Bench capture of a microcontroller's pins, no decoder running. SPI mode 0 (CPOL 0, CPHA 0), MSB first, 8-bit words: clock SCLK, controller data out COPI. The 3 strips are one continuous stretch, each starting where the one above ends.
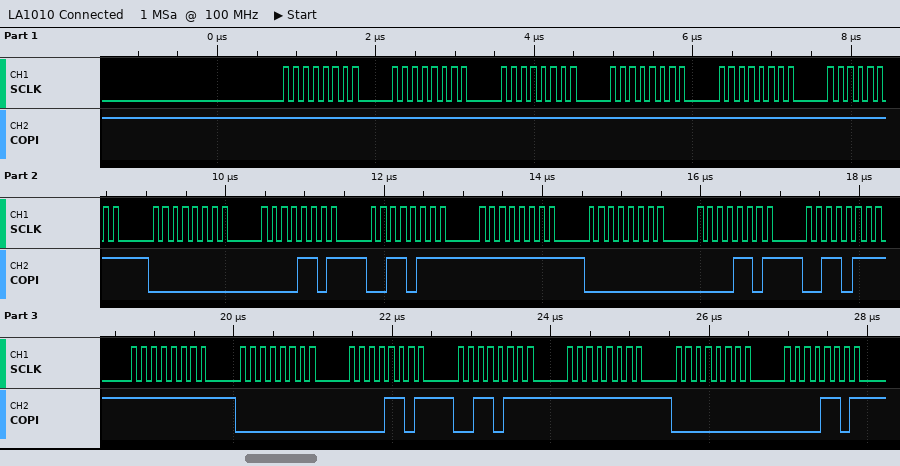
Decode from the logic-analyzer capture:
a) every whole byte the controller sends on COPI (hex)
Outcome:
0xFF 0xFF 0xFF 0xFF 0xFF 0xFF 0x00 0x0D 0x37 0xFF 0x00 0x0D 0x37 0xFF 0x00 0x0D 0x37 0xFF 0x00 0x0D
